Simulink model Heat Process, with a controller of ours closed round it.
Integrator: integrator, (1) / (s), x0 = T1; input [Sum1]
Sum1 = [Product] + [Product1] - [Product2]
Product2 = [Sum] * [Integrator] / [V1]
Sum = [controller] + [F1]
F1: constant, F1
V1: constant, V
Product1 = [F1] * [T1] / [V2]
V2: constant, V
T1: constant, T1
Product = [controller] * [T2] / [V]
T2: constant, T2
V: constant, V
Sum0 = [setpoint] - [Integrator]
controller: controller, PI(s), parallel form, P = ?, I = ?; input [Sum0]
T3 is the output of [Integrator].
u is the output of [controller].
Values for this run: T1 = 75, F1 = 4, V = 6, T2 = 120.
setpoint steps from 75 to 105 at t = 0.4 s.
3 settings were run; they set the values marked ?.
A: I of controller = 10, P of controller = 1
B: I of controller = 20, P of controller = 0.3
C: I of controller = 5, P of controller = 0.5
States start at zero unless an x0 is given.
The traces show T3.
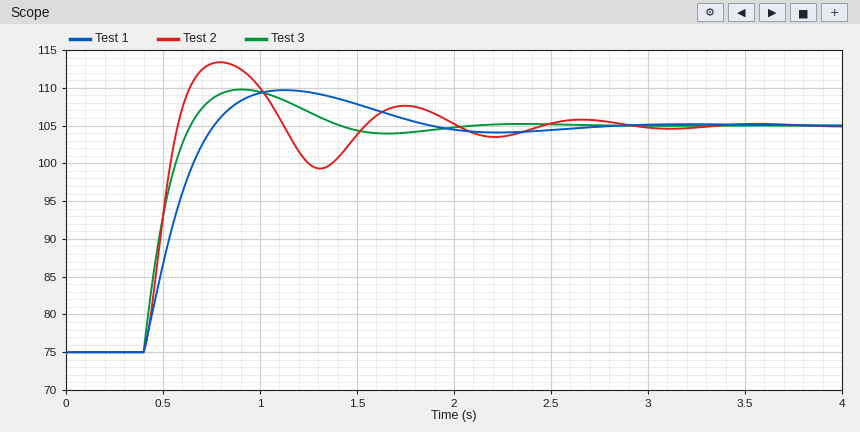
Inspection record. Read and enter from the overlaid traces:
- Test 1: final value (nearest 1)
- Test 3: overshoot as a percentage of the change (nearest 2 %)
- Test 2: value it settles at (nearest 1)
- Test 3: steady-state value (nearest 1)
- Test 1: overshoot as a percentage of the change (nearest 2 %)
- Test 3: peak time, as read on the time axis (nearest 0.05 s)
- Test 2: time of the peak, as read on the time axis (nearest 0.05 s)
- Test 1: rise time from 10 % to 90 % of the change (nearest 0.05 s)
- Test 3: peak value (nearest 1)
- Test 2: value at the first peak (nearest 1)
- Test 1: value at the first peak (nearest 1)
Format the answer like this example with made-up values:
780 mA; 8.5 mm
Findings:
105; 16 %; 105; 105; 16 %; 0.90 s; 0.80 s; 0.25 s; 110; 113; 110
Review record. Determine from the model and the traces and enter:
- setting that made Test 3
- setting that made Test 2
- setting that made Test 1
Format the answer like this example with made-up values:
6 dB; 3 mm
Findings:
A; B; C
